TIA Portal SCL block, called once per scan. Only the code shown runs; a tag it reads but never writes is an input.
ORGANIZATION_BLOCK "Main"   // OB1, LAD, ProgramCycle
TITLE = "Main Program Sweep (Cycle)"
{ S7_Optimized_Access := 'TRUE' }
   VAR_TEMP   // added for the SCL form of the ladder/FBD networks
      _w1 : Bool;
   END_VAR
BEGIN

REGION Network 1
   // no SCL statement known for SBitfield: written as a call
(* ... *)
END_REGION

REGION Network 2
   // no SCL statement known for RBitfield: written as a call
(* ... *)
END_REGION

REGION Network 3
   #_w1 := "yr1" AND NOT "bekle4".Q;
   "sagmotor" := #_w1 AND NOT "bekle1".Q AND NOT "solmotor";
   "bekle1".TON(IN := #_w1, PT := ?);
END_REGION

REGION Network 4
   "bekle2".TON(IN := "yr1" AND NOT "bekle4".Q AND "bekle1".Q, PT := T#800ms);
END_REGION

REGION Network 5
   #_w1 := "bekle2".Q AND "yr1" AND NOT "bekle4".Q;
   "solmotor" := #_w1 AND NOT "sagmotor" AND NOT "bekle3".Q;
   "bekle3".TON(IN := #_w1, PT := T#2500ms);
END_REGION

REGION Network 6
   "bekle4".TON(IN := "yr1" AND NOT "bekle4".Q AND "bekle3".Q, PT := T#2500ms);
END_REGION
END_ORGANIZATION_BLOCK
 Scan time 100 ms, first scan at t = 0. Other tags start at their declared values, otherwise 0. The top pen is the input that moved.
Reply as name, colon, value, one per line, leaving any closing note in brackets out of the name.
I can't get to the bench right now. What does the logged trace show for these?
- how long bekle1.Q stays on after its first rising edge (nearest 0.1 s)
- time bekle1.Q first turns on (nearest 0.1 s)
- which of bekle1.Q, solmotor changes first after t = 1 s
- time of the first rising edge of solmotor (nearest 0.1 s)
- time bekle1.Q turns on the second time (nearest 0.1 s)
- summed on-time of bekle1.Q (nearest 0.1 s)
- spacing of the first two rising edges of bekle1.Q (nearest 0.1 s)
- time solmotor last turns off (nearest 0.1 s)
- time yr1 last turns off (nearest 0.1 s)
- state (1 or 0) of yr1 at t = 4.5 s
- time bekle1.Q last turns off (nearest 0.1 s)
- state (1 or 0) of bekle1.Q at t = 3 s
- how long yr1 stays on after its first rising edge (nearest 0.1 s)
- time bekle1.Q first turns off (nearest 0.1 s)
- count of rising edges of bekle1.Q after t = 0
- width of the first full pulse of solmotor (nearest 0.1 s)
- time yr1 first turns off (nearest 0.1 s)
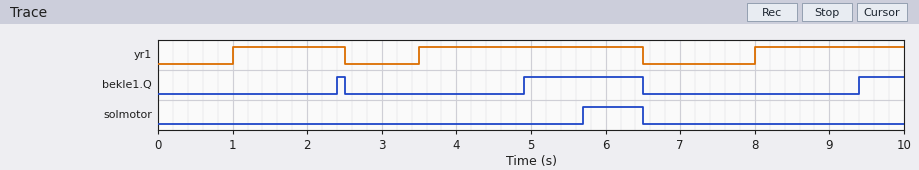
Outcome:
how long bekle1.Q stays on after its first rising edge: 0.1 s
time bekle1.Q first turns on: 2.4 s
which of bekle1.Q, solmotor changes first after t = 1 s: bekle1.Q
time of the first rising edge of solmotor: 5.7 s
time bekle1.Q turns on the second time: 4.9 s
summed on-time of bekle1.Q: 2.3 s
spacing of the first two rising edges of bekle1.Q: 2.5 s
time solmotor last turns off: 6.5 s
time yr1 last turns off: 6.5 s
state (1 or 0) of yr1 at t = 4.5 s: 1
time bekle1.Q last turns off: 6.5 s
state (1 or 0) of bekle1.Q at t = 3 s: 0
how long yr1 stays on after its first rising edge: 1.5 s
time bekle1.Q first turns off: 2.5 s
count of rising edges of bekle1.Q after t = 0: 3
width of the first full pulse of solmotor: 0.8 s
time yr1 first turns off: 2.5 s
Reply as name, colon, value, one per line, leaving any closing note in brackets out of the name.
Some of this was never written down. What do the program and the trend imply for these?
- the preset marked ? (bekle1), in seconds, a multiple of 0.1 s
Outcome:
the preset marked ? (bekle1), in seconds, a multiple of 0.1 s: 1.4 s
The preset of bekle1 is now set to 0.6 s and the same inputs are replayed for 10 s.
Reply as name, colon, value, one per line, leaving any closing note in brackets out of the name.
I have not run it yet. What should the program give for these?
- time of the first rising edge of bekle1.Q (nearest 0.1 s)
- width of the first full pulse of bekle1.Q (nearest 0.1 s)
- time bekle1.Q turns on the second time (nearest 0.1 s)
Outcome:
time of the first rising edge of bekle1.Q: 1.6 s
width of the first full pulse of bekle1.Q: 0.9 s
time bekle1.Q turns on the second time: 4.1 s
